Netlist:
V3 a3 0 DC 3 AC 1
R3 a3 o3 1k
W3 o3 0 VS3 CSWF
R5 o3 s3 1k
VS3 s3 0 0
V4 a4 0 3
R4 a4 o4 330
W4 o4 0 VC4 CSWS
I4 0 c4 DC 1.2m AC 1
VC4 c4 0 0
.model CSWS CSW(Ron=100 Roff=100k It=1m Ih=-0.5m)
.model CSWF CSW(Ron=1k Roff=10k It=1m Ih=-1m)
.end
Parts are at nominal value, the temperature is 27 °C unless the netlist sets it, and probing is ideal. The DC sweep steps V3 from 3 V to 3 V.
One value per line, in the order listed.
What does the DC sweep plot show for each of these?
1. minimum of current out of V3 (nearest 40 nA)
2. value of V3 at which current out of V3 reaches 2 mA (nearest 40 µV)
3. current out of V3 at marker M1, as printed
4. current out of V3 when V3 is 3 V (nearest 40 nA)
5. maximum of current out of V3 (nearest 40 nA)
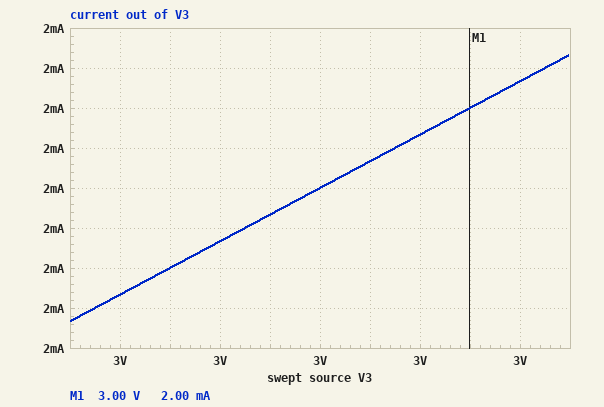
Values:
1.99932 mA
3.00000 V
2.00 mA
1.99960 mA
2.00068 mA
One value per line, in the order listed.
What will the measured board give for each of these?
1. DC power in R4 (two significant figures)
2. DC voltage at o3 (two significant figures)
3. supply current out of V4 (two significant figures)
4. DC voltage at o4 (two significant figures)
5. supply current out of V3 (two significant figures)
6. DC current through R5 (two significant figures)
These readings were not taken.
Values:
16 mW
1.0 V
7.0 mA
700 mV
2.0 mA
1.0 mA
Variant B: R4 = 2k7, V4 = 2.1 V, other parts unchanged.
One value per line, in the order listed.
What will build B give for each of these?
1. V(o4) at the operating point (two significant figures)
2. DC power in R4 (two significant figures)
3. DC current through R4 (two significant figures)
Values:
75 mV
1.5 mW
750 µA
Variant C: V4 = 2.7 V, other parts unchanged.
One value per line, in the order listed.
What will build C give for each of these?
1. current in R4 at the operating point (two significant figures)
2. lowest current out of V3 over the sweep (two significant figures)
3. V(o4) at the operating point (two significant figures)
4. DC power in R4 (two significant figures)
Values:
6.3 mA
2.0 mA
630 mV
13 mW
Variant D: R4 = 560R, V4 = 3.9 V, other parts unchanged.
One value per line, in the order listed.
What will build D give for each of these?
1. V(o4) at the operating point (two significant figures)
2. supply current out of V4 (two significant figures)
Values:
590 mV
5.9 mA
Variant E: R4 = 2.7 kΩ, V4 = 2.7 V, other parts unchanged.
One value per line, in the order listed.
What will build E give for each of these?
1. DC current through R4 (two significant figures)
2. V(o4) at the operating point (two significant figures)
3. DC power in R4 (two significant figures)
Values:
960 µA
96 mV
2.5 mW
